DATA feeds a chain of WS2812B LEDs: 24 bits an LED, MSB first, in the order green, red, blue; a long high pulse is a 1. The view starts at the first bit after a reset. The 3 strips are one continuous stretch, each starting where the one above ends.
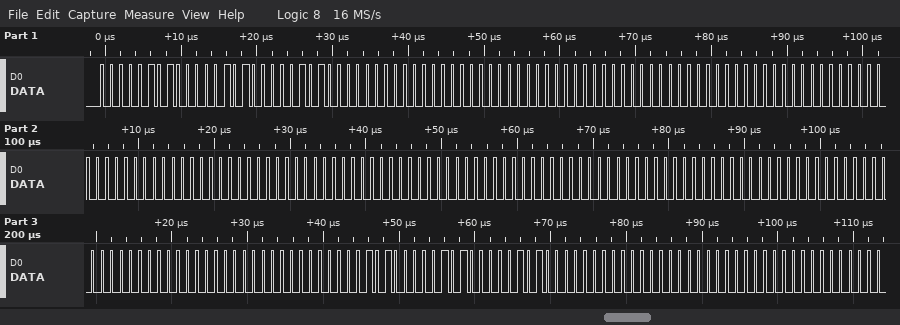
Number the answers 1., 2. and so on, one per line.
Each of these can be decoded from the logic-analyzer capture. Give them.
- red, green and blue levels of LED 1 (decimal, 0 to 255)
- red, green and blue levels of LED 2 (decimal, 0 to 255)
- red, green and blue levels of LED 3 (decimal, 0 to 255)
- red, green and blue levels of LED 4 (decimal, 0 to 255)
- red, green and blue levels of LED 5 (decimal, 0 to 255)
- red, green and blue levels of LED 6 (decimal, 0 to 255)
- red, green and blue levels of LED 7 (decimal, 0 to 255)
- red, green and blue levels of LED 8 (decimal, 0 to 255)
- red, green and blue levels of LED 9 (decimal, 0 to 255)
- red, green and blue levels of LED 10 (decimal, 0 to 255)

1. 5, 5, 5
2. 0, 0, 0
3. 0, 0, 0
4. 0, 0, 0
5. 0, 0, 0
6. 0, 0, 0
7. 0, 0, 0
8. 0, 0, 0
9. 5, 5, 5
10. 0, 0, 0
